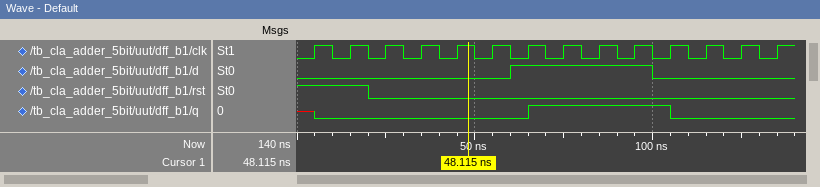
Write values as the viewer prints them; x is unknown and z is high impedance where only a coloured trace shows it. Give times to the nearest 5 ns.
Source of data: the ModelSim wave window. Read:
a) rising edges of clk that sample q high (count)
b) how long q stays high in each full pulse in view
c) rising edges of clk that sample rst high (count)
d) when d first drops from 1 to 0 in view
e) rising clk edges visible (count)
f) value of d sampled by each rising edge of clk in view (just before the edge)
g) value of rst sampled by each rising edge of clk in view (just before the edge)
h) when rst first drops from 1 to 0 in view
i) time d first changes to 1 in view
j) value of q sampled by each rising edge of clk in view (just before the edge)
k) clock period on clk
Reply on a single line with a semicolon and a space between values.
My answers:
4; 40 ns; 2; 100 ns; 14; 0 0 0 0 0 0 1 1 1 1 0 0 0 0; 1 1 0 0 0 0 0 0 0 0 0 0 0 0; 20 ns; 60 ns; x 0 0 0 0 0 0 1 1 1 1 0 0 0; 10 ns
